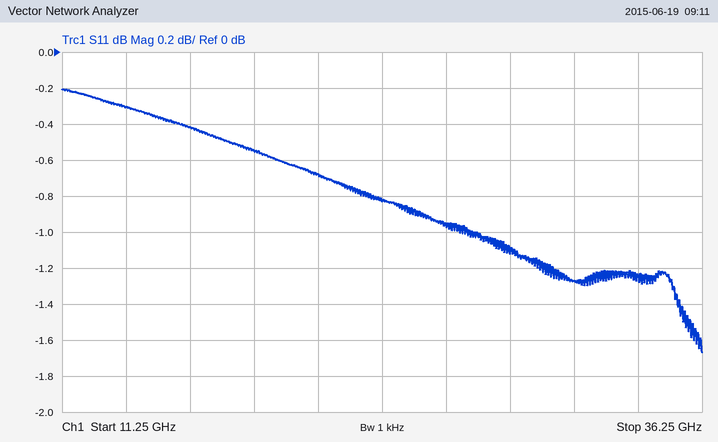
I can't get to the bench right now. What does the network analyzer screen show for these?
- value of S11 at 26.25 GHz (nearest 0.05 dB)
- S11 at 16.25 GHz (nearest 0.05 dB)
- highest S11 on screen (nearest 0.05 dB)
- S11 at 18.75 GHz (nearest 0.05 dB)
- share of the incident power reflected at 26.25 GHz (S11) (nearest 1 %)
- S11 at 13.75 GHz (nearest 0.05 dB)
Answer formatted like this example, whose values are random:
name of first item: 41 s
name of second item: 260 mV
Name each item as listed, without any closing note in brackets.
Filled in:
value of S11 at 26.25 GHz: -0.95 dB
S11 at 16.25 GHz: -0.40 dB
highest S11 on screen: -0.20 dB
S11 at 18.75 GHz: -0.55 dB
share of the incident power reflected at 26.25 GHz (S11): 80 %
S11 at 13.75 GHz: -0.30 dB
